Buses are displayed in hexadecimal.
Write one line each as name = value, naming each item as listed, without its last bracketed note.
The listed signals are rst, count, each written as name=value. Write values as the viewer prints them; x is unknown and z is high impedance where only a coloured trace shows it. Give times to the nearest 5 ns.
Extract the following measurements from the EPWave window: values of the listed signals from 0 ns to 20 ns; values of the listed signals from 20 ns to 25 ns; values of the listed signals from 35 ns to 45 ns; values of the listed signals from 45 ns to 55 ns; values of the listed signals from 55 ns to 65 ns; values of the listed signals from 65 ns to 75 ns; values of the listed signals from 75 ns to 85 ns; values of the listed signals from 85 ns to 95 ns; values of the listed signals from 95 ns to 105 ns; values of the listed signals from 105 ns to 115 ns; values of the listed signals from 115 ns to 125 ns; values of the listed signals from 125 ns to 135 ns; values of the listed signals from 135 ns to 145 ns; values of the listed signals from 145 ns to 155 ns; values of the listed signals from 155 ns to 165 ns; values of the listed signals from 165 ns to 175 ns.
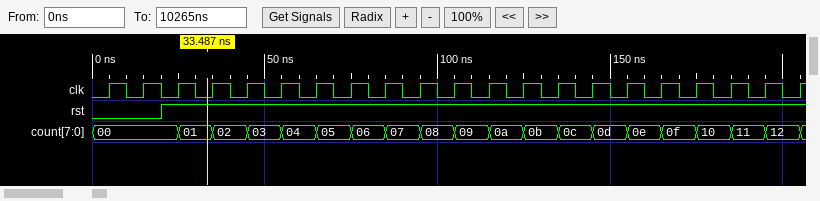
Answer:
values of the listed signals from 0 ns to 20 ns = rst=0, count=00
values of the listed signals from 20 ns to 25 ns = rst=1, count=00
values of the listed signals from 35 ns to 45 ns = rst=1, count=02
values of the listed signals from 45 ns to 55 ns = rst=1, count=03
values of the listed signals from 55 ns to 65 ns = rst=1, count=04
values of the listed signals from 65 ns to 75 ns = rst=1, count=05
values of the listed signals from 75 ns to 85 ns = rst=1, count=06
values of the listed signals from 85 ns to 95 ns = rst=1, count=07
values of the listed signals from 95 ns to 105 ns = rst=1, count=08
values of the listed signals from 105 ns to 115 ns = rst=1, count=09
values of the listed signals from 115 ns to 125 ns = rst=1, count=0a
values of the listed signals from 125 ns to 135 ns = rst=1, count=0b
values of the listed signals from 135 ns to 145 ns = rst=1, count=0c
values of the listed signals from 145 ns to 155 ns = rst=1, count=0d
values of the listed signals from 155 ns to 165 ns = rst=1, count=0e
values of the listed signals from 165 ns to 175 ns = rst=1, count=0f
